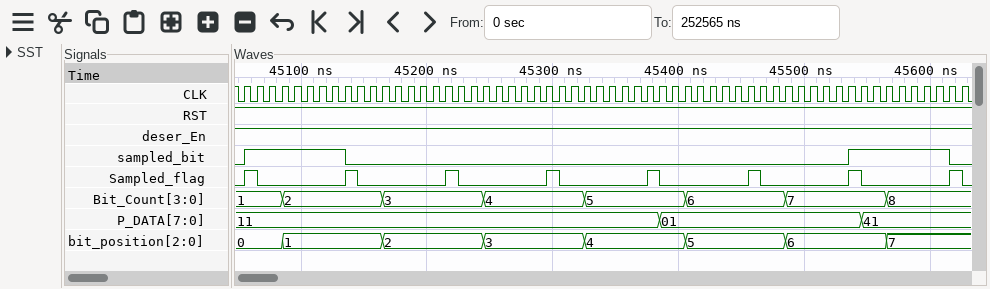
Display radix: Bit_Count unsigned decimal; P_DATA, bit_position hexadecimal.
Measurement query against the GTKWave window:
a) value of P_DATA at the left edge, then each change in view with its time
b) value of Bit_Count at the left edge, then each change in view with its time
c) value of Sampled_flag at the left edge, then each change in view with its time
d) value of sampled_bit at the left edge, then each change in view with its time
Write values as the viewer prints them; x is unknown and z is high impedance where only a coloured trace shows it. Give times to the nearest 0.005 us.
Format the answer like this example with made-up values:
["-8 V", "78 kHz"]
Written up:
["11, 01 at 45.385 us, 41 at 45.545 us", "1, 2 at 45.085 us, 3 at 45.165 us, 4 at 45.245 us, 5 at 45.325 us, 6 at 45.405 us, 7 at 45.485 us, 8 at 45.565 us", "0, 1 at 45.055 us, 0 at 45.065 us, 1 at 45.135 us, 0 at 45.145 us, 1 at 45.215 us, 0 at 45.225 us, 1 at 45.295 us, 0 at 45.305 us, 1 at 45.375 us, 0 at 45.385 us, 1 at 45.455 us, 0 at 45.465 us, 1 at 45.535 us, 0 at 45.545 us, 1 at 45.615 us, 0 at 45.625 us", "0, 1 at 45.055 us, 0 at 45.135 us, 1 at 45.535 us, 0 at 45.615 us"]
